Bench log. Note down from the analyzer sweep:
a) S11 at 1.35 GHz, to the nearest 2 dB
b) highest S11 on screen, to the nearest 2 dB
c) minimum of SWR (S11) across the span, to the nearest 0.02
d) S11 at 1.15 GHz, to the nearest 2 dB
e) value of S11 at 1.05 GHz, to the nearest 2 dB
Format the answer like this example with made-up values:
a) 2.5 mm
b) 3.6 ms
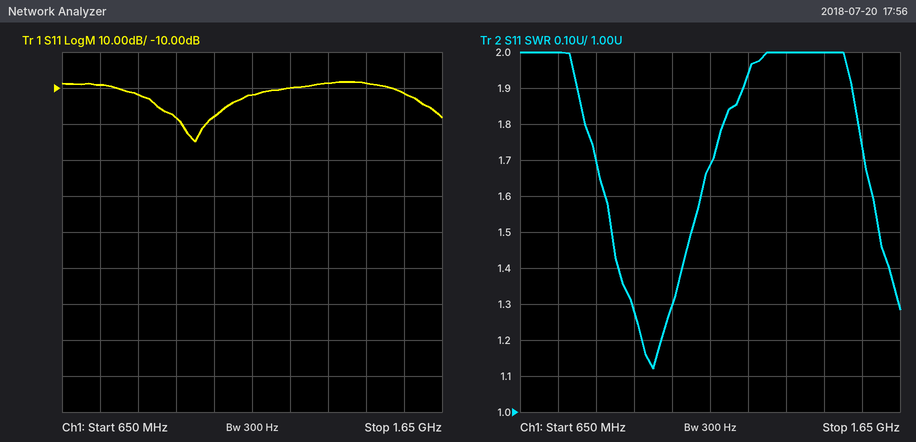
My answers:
a) -8 dB
b) -8 dB
c) 1.12
d) -12 dB
e) -18 dB
